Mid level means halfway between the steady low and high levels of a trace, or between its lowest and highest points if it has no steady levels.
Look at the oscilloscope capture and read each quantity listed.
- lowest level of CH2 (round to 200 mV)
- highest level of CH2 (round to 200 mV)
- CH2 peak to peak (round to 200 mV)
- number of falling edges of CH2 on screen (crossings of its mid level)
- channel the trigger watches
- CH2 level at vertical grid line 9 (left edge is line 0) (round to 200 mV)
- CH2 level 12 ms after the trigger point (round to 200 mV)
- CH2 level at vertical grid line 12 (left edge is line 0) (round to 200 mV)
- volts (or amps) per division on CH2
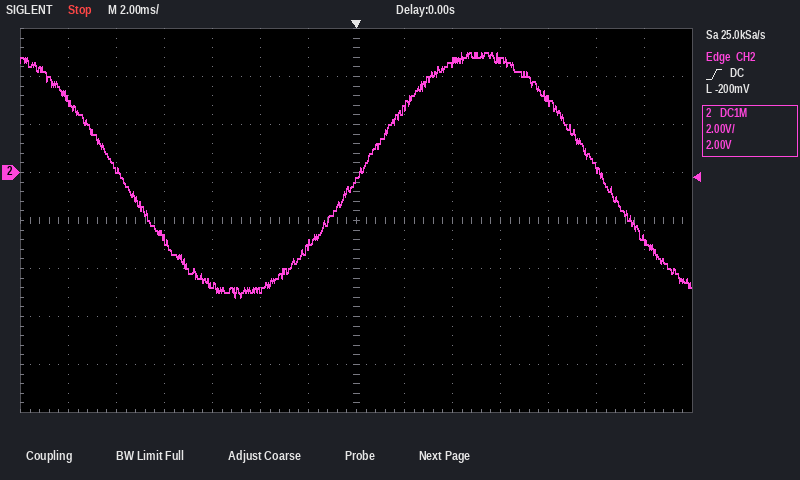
-5.2 V
5.0 V
10.2 V
2
CH2
4.6 V
-2.8 V
200 mV
2 V
